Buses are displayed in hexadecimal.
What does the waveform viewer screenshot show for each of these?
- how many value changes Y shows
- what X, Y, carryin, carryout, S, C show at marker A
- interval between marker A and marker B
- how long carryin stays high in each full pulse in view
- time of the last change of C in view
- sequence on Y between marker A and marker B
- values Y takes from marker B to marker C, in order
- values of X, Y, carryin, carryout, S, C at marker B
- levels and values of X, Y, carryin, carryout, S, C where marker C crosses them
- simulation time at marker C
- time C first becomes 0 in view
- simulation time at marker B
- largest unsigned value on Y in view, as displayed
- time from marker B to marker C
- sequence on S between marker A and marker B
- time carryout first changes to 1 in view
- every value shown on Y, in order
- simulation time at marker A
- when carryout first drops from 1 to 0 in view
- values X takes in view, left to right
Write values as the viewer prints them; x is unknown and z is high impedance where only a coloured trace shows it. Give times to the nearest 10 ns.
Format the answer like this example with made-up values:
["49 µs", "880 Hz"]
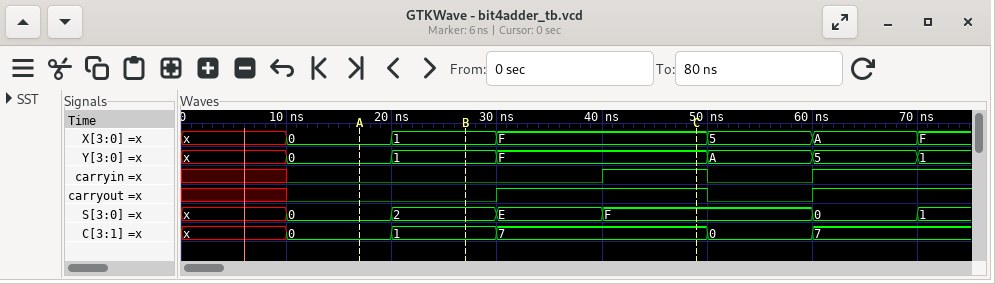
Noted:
["6", "X=0, Y=0, carryin=0, carryout=0, S=0, C=0", "10 ns", "10 ns", "60 ns", "0, 1", "1, F", "X=1, Y=1, carryin=0, carryout=0, S=2, C=1", "X=F, Y=F, carryin=1, carryout=1, S=F, C=7", "50 ns", "10 ns", "30 ns", "F", "20 ns", "0, 2", "30 ns", "x, 0, 1, F, A, 5, 1", "20 ns", "50 ns", "x, 0, 1, F, 5, A, F"]
